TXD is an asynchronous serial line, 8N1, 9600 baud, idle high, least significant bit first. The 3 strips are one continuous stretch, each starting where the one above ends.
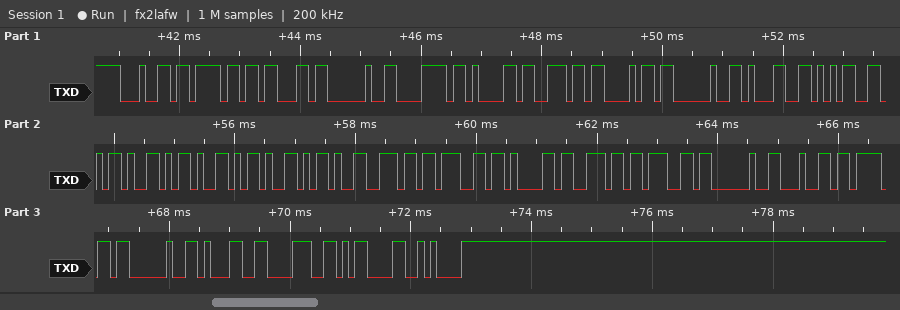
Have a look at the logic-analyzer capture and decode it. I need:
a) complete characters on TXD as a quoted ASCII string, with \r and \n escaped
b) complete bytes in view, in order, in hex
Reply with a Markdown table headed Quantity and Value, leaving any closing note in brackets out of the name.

| Quantity | Value |
|---|---|
| complete characters on TXD as a quoted ASCII string, with \r and \n escaped | "doc xanh 15----ngang do 18\r\n" |
| complete bytes in view, in order, in hex | 64 6F 63 20 78 61 6E 68 20 31 35 2D 2D 2D 2D 6E 67 61 6E 67 20 64 6F 20 31 38 0D 0A |
